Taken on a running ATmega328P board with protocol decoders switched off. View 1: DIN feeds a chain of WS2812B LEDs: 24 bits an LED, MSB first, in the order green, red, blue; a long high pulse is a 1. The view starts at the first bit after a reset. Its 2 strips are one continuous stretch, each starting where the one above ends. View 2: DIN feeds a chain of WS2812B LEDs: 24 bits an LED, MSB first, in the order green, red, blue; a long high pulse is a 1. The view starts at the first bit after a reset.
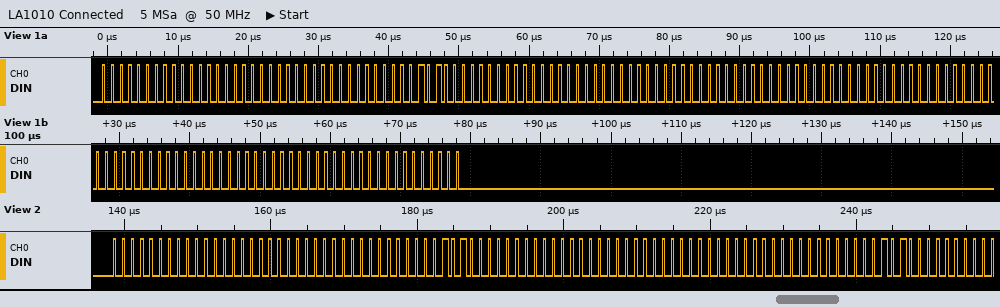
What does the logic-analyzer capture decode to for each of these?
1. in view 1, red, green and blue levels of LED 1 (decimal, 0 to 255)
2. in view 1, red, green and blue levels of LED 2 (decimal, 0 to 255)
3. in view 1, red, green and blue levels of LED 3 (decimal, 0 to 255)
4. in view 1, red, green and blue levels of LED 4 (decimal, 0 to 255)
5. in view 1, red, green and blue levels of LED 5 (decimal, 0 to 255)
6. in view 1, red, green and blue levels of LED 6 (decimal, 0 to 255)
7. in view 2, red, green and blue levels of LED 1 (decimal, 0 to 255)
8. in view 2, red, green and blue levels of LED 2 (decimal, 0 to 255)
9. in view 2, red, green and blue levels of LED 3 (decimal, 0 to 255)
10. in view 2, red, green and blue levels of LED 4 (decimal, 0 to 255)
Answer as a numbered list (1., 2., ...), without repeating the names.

1. 0, 0, 0
2. 10, 0, 0
3. 0, 0, 0
4. 0, 0, 0
5. 0, 0, 0
6. 0, 0, 0
7. 0, 0, 0
8. 10, 0, 0
9. 0, 0, 0
10. 10, 0, 0
